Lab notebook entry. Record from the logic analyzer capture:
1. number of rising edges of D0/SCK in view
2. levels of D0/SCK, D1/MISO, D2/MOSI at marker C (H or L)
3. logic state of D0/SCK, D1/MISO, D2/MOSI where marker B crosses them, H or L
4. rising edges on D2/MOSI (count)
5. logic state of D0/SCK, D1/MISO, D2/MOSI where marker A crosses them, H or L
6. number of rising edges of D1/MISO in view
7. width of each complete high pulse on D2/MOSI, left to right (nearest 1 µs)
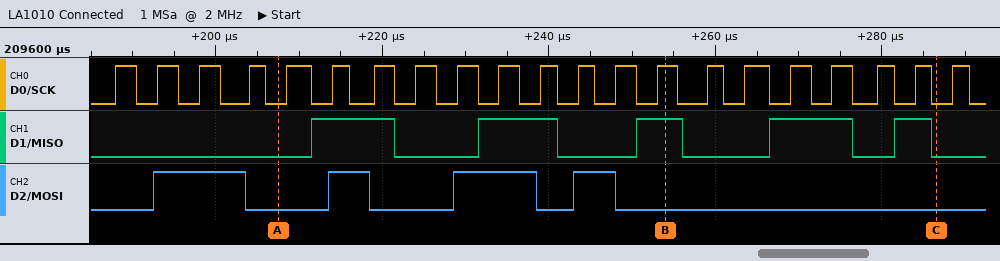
21
D0/SCK=L, D1/MISO=L, D2/MOSI=L
D0/SCK=H, D1/MISO=H, D2/MOSI=L
4
D0/SCK=L, D1/MISO=L, D2/MOSI=L
5
11 µs, 5 µs, 10 µs, 5 µs
